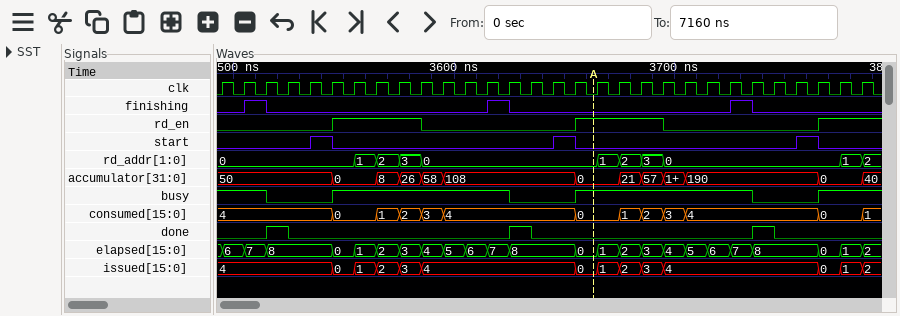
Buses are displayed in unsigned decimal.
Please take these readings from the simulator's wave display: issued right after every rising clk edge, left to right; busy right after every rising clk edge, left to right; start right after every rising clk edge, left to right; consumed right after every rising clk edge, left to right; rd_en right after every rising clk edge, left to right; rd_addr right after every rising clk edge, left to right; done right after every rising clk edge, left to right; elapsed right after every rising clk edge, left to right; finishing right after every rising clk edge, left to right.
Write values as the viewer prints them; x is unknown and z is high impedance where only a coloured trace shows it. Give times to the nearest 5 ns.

4, 4, 4, 4, 4, 0, 1, 2, 3, 4, 4, 4, 4, 4, 4, 4, 0, 1, 2, 3, 4, 4, 4, 4, 4, 4, 4, 0, 1, 2
1 1 0 0 0 1 1 1 1 1 1 1 1 0 0 0 1 1 1 1 1 1 1 1 0 0 0 1 1 1
0 0 0 0 1 0 0 0 0 0 0 0 0 0 0 1 0 0 0 0 0 0 0 0 0 0 1 0 0 0
4, 4, 4, 4, 4, 0, 0, 1, 2, 3, 4, 4, 4, 4, 4, 4, 0, 0, 1, 2, 3, 4, 4, 4, 4, 4, 4, 0, 0, 1
0 0 0 0 0 1 1 1 1 0 0 0 0 0 0 0 1 1 1 1 0 0 0 0 0 0 0 1 1 1
0, 0, 0, 0, 0, 0, 1, 2, 3, 0, 0, 0, 0, 0, 0, 0, 0, 1, 2, 3, 0, 0, 0, 0, 0, 0, 0, 0, 1, 2
0 0 1 0 0 0 0 0 0 0 0 0 0 1 0 0 0 0 0 0 0 0 0 0 1 0 0 0 0 0
6, 7, 8, 8, 8, 0, 1, 2, 3, 4, 5, 6, 7, 8, 8, 8, 0, 1, 2, 3, 4, 5, 6, 7, 8, 8, 8, 0, 1, 2
0 1 0 0 0 0 0 0 0 0 0 0 1 0 0 0 0 0 0 0 0 0 0 1 0 0 0 0 0 0
